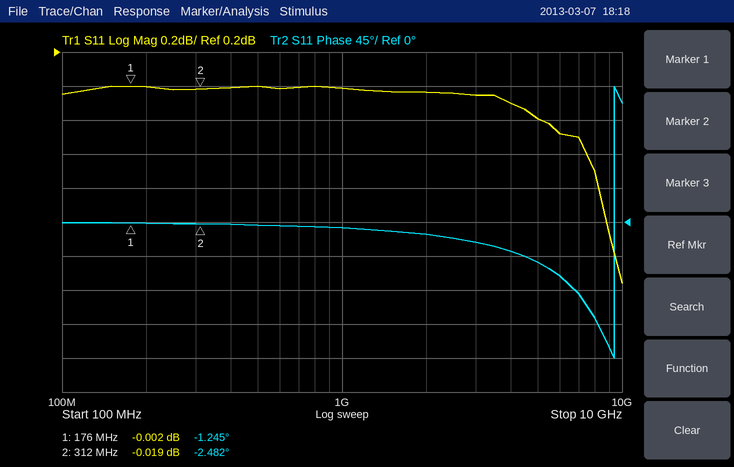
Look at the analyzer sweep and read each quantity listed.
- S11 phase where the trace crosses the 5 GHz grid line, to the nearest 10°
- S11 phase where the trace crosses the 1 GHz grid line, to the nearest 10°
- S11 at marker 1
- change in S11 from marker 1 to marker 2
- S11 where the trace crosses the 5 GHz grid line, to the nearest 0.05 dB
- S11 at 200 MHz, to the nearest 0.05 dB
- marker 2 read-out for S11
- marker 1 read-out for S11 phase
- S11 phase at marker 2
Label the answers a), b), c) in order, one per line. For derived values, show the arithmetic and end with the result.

a) -50°
b) -10°
c) -0.002 dB
d) -0.019 − (-0.002) = -0.017 dB
e) -0.20 dB
f) 0.00 dB
g) -0.019 dB
h) -1.245°
i) -2.482°
